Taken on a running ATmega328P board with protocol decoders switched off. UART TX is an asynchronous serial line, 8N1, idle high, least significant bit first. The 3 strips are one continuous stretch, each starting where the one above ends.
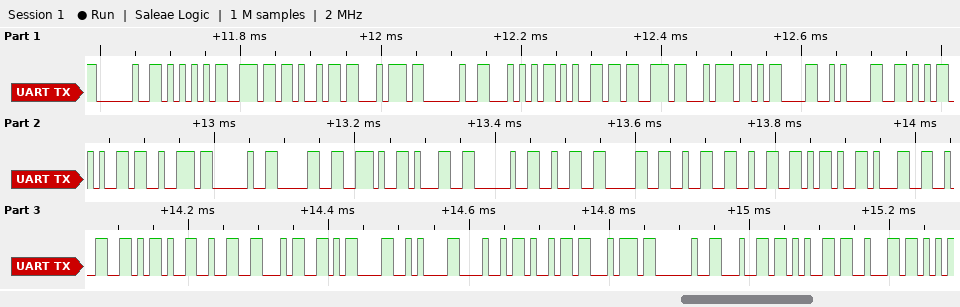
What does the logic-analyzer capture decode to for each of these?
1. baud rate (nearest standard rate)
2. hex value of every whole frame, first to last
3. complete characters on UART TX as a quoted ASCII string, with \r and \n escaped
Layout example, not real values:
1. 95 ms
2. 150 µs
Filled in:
1. 115200 baud
2. 20 55 6E 69 74 20 54 65 73 74 0D 0A 56 65 72 20 30 2E 31 20 32 30 32 32 2D 31 32 2D 32 34 0D 0A 48 69 74 20 64 65 62
3. " Unit Test\r\nVer 0.1 2022-12-24\r\nHit deb"
